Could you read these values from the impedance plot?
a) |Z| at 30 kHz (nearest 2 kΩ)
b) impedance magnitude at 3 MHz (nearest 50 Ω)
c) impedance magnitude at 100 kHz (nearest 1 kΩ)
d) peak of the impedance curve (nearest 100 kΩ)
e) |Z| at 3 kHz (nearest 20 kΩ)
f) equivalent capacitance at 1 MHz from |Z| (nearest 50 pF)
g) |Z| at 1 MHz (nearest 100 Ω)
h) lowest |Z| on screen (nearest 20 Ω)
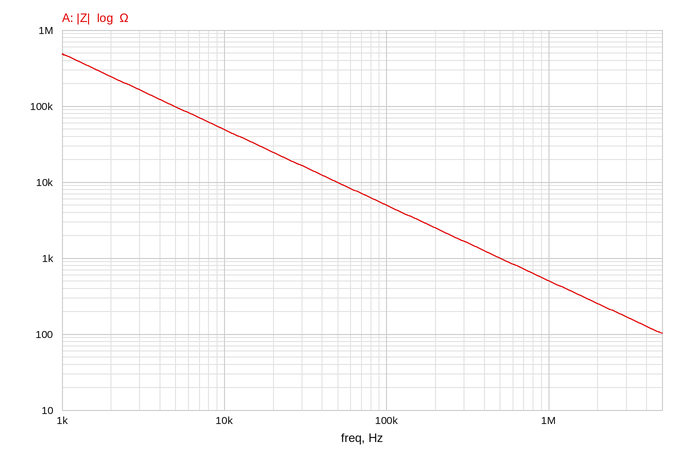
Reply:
16 kΩ
150 Ω
5 kΩ
500 kΩ
160 kΩ
300 pF
500 Ω
100 Ω
